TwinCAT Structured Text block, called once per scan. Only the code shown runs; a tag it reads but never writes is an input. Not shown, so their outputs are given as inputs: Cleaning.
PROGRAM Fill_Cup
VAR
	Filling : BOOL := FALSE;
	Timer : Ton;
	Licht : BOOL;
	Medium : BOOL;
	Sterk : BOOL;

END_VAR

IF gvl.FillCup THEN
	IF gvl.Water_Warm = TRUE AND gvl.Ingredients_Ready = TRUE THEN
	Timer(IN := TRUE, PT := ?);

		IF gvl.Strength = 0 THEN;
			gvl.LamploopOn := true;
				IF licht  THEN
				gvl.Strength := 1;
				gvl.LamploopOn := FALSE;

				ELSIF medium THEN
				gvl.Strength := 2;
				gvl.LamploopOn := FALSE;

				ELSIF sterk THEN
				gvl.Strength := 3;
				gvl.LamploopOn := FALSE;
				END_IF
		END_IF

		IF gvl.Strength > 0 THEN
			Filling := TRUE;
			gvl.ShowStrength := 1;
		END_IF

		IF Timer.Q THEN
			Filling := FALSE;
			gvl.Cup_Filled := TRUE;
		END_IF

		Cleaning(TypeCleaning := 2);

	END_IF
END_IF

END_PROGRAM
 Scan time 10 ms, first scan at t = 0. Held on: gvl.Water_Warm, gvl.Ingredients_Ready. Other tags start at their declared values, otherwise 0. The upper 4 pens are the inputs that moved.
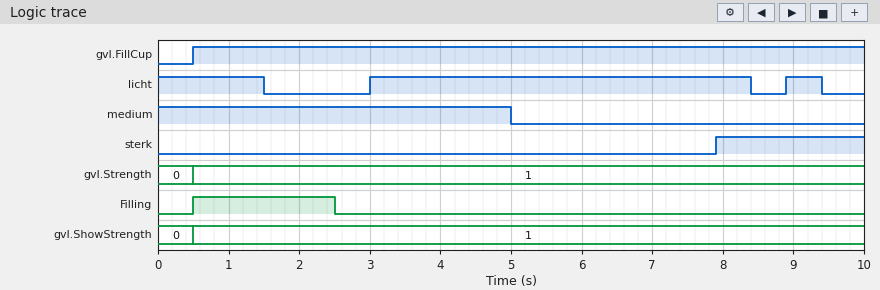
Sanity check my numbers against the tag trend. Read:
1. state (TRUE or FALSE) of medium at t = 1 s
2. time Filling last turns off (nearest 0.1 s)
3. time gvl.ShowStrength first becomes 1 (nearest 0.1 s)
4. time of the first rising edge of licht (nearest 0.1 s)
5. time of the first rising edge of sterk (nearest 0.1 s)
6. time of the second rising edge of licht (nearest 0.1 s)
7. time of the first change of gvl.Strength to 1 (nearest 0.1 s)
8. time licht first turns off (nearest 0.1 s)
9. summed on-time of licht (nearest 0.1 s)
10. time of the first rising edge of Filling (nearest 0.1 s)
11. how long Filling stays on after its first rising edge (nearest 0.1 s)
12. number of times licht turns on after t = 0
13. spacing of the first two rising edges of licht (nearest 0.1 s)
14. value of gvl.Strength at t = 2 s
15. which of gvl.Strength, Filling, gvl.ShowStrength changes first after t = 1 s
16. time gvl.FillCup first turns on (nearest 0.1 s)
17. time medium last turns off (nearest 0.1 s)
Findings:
TRUE
2.5 s
0.5 s
3.0 s
7.9 s
8.9 s
0.5 s
1.5 s
7.4 s
0.5 s
2.0 s
2
5.9 s
1
Filling
0.5 s
5.0 s
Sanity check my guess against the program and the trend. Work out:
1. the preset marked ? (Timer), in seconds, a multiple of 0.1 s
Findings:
2.0 s
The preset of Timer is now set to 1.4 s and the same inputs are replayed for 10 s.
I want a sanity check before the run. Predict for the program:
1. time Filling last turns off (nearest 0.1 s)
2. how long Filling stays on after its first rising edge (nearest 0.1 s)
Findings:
1.9 s
1.4 s
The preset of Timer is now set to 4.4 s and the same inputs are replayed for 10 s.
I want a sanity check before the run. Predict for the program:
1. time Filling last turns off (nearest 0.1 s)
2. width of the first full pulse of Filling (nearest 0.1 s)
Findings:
4.9 s
4.4 s
